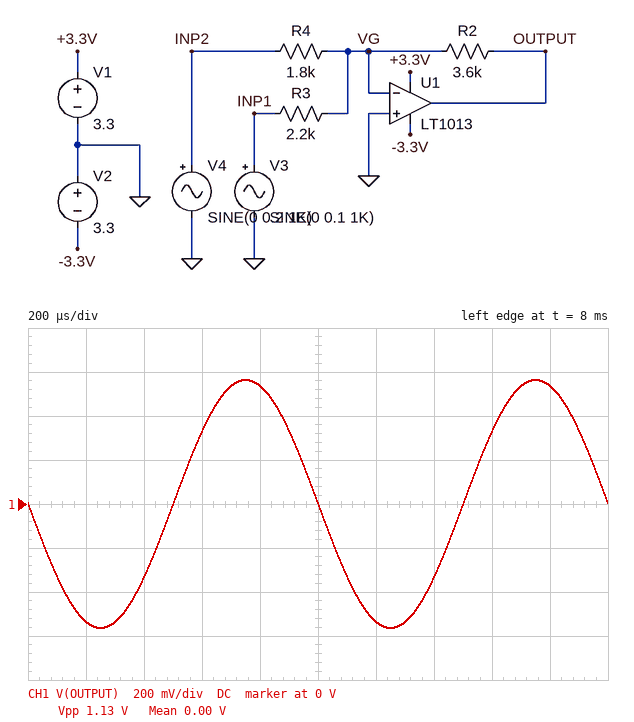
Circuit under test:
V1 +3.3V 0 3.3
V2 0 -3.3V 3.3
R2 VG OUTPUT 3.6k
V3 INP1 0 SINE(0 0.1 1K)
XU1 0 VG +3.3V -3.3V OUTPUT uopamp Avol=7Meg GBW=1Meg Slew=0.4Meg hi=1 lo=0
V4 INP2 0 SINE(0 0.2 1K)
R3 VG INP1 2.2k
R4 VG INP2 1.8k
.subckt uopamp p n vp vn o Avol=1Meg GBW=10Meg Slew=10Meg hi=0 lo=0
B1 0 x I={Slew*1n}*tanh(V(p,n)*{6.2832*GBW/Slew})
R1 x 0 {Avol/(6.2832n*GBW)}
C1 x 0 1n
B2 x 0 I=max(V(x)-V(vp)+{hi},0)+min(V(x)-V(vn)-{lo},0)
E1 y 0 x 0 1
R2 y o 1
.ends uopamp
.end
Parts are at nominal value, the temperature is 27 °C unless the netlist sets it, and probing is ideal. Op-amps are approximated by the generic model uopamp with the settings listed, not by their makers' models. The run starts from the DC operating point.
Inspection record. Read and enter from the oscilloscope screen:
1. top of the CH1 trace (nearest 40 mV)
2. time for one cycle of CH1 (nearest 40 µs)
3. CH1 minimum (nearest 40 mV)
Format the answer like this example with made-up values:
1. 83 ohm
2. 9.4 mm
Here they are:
1. 560 mV
2. 1.00 ms
3. -560 mV
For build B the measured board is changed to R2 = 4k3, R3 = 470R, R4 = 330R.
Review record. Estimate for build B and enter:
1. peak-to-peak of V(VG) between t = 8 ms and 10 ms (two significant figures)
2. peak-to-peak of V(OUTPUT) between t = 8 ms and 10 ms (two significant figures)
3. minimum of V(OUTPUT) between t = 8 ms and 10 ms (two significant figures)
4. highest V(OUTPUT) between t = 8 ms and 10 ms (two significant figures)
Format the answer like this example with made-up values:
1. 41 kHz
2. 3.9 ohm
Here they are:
1. 62 mV
2. 5.6 V
3. -3.3 V
4. 2.3 V
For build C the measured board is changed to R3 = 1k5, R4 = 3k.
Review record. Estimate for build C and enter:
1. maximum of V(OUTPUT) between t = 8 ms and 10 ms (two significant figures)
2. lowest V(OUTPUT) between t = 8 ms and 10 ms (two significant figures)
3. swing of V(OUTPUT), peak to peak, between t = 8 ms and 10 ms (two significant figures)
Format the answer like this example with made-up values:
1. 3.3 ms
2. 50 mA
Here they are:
1. 480 mV
2. -480 mV
3. 960 mV
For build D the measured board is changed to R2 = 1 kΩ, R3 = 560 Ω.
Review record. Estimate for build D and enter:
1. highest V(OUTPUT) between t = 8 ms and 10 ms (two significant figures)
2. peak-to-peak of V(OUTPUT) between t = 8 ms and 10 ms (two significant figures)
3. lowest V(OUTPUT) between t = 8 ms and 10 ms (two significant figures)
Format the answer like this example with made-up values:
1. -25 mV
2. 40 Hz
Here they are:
1. 290 mV
2. 580 mV
3. -290 mV
